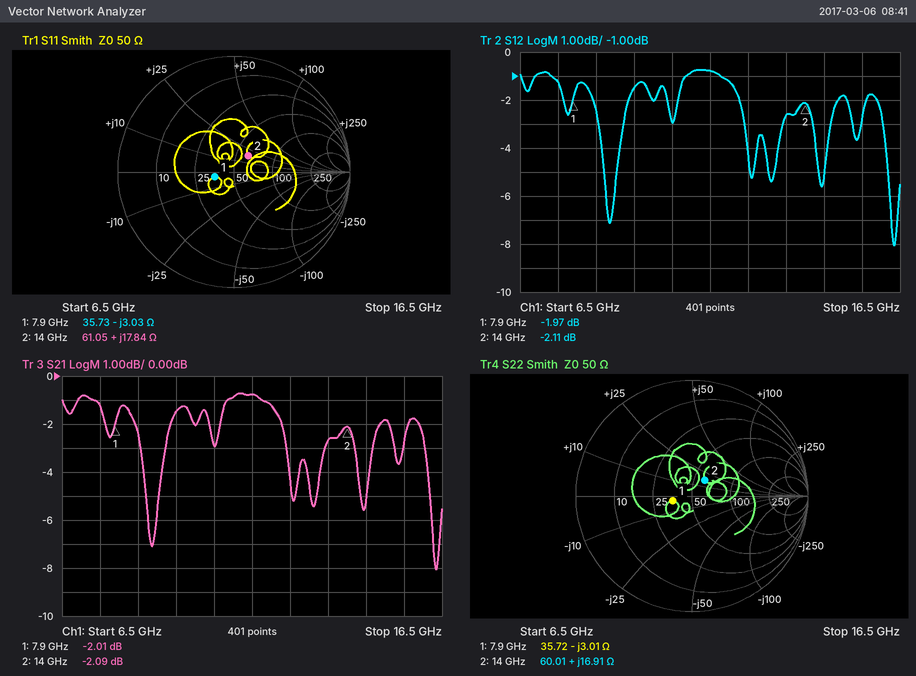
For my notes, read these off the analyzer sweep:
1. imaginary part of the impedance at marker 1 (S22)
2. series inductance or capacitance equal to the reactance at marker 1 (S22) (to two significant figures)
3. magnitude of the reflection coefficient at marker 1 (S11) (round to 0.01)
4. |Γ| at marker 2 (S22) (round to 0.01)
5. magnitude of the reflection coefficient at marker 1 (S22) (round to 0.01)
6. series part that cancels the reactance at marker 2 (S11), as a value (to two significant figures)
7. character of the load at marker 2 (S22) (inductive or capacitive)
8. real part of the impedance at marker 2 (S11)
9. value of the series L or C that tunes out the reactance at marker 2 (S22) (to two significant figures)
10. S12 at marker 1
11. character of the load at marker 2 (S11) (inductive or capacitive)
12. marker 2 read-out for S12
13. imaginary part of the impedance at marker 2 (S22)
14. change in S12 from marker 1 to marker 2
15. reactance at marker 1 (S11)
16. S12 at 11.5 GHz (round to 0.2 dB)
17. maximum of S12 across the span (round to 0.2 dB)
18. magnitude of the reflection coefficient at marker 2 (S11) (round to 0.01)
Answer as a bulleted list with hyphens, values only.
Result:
- -3.01 Ω
- 6.7 pF
- 0.17
- 0.18
- 0.17
- 640 fF
- inductive
- 61.05 Ω
- 670 fF
- -1.97 dB
- inductive
- -2.11 dB
- +16.91 Ω
- -0.14 dB
- -3.03 Ω
- -0.8 dB
- -0.8 dB
- 0.19
